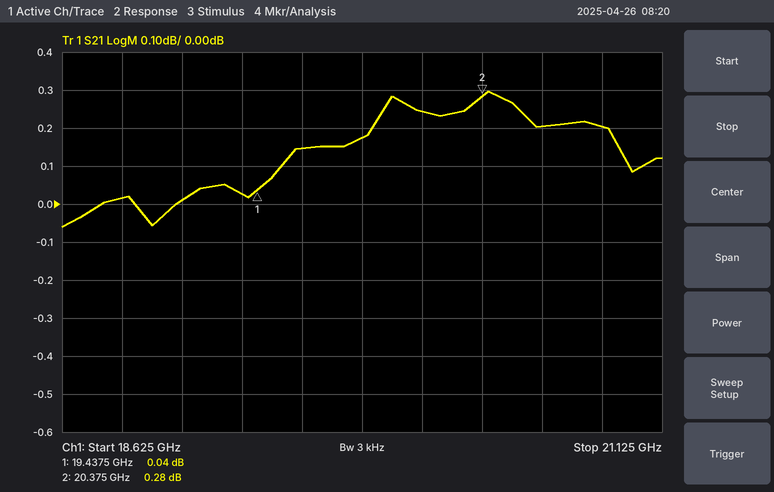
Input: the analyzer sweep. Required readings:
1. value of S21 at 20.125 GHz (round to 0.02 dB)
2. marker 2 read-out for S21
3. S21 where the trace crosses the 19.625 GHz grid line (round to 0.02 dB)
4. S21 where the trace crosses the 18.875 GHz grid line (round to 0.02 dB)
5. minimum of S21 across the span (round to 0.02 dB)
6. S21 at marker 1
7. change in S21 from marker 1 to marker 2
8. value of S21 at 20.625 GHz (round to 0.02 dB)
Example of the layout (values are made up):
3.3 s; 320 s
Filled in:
0.24 dB; 0.28 dB; 0.14 dB; 0.02 dB; -0.06 dB; 0.04 dB; 0.24 dB; 0.20 dB
